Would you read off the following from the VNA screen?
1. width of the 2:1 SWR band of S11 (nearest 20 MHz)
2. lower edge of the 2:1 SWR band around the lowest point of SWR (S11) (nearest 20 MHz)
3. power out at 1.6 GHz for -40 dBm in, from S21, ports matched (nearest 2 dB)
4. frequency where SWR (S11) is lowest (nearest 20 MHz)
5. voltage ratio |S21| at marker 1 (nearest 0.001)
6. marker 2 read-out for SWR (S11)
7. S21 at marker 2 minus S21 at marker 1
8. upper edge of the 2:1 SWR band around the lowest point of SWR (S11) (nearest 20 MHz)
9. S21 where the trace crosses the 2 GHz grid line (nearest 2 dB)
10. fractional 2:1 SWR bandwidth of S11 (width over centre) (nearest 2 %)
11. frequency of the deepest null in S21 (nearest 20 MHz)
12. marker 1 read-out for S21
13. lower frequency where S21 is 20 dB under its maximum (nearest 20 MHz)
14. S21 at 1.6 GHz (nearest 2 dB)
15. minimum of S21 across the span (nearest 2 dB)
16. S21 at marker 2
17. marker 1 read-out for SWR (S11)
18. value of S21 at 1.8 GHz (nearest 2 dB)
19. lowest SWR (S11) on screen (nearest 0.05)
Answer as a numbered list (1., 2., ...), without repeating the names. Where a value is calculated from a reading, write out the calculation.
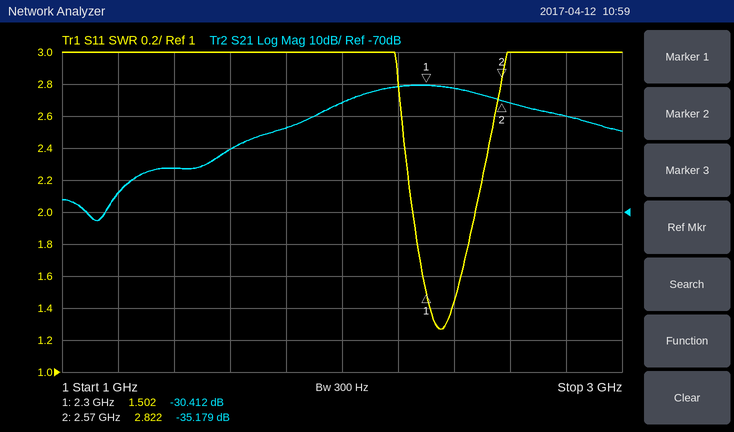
1. 2.48 GHz − 2.26 GHz = 220 MHz
2. 2.26 GHz
3. -40 dBm + (-50 dB) = -90 dBm
4. 2.36 GHz
5. 10^(-30.412/20) ≈ 0.030
6. 2.822
7. -35.179 − (-30.412) = -4.767 dB
8. 2.48 GHz
9. -36 dB
10. 220 MHz / 2.37 GHz ≈ 9.28 %, so 10 % to the nearest 2 %
11. 1.12 GHz
12. -30.412 dB
13. 1.60 GHz
14. -50 dB
15. -72 dB
16. -35.179 dB
17. 1.502
18. -44 dB
19. 1.25
